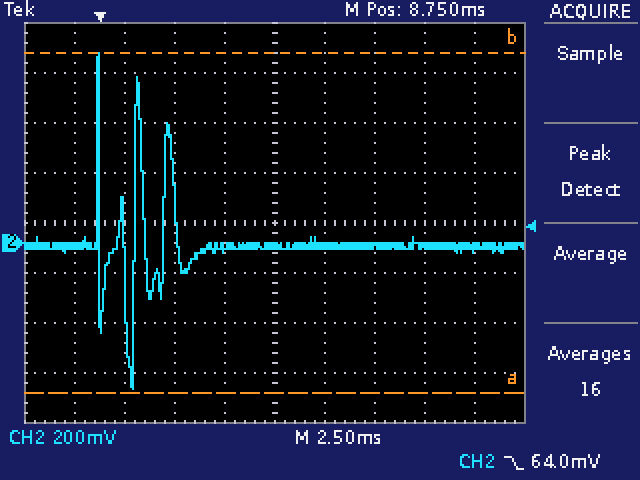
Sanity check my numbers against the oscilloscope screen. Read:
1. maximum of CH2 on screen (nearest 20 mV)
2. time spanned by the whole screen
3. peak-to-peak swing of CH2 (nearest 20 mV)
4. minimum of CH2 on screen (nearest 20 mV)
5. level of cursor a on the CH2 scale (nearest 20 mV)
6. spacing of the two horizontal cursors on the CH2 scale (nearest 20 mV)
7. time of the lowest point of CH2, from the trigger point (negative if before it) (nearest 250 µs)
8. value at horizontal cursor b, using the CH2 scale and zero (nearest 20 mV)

760 mV
25 ms
1.34 V
-580 mV
-600 mV
1.36 V
+1.75 ms
760 mV
